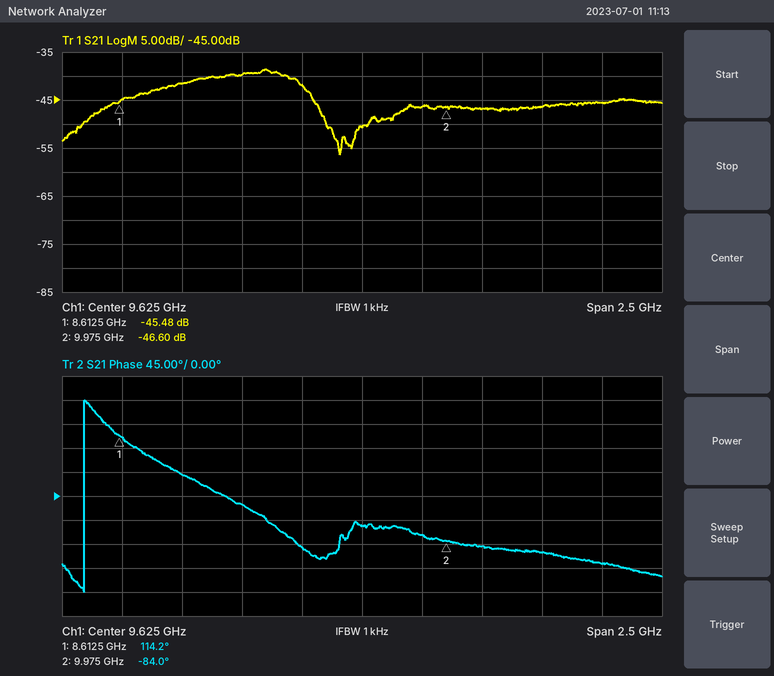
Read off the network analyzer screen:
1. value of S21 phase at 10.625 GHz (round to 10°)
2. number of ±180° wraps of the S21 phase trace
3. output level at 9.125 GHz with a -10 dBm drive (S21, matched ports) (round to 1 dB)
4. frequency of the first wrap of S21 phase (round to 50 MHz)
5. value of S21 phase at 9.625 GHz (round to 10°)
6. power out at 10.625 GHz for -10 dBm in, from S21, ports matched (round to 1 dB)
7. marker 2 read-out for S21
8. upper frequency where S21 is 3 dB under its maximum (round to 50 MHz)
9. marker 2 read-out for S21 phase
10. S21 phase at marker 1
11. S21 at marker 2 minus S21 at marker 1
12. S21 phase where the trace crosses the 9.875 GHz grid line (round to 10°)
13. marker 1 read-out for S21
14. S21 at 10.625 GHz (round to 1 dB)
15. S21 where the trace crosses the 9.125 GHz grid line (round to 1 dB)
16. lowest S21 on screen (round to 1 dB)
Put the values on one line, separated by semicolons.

-130°; 1; -50 dBm; 8.45 GHz; -60°; -56 dBm; -46.60 dB; 9.35 GHz; -84.0°; 114.2°; -1.12 dB; -70°; -45.48 dB; -46 dB; -40 dB; -56 dB
